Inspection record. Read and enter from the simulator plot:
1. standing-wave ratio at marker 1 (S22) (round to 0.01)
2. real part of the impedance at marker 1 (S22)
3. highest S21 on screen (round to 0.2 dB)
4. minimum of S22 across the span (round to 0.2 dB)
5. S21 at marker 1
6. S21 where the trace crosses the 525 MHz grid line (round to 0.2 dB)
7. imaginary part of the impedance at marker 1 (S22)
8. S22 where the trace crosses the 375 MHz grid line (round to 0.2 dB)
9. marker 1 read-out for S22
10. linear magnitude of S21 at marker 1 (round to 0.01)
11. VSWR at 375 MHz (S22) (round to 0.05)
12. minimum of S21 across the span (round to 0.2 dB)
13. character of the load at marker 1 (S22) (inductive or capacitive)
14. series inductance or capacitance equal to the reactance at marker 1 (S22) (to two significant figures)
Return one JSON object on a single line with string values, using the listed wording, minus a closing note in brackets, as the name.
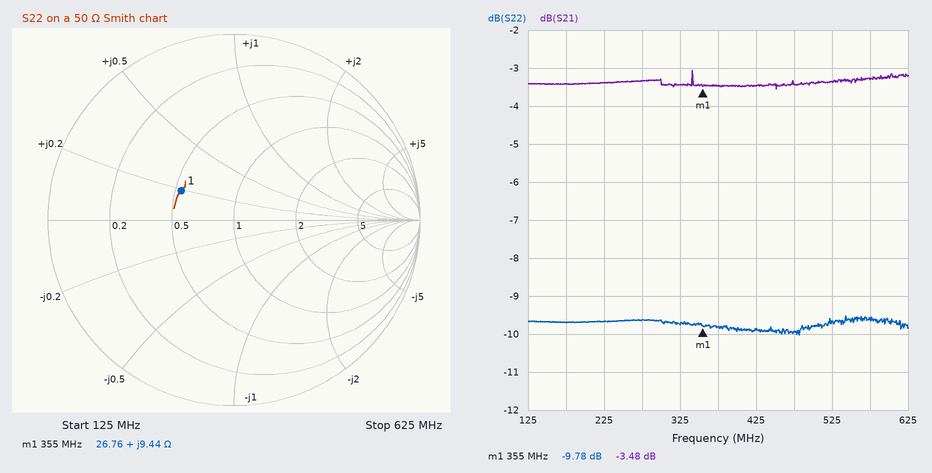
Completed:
{"standing-wave ratio at marker 1 (S22)": "1.96", "real part of the impedance at marker 1": "26.76 Ω", "highest S21 on screen": "-3.0 dB", "minimum of S22 across the span": "-10.0 dB", "S21 at marker 1": "-3.48 dB", "S21 where the trace crosses the 525 MHz grid line": "-3.4 dB", "imaginary part of the impedance at marker 1": "+9.44 Ω", "S22 where the trace crosses the 375 MHz grid line": "-9.8 dB", "marker 1 read-out for S22": "-9.78 dB", "linear magnitude of S21 at marker 1": "0.67", "VSWR at 375 MHz (S22)": "1.95", "minimum of S21 across the span": "-3.6 dB", "character of the load at marker 1 (S22)": "inductive", "series inductance or capacitance equal to the reactance at marker 1 (S22)": "4.2 nH"}
